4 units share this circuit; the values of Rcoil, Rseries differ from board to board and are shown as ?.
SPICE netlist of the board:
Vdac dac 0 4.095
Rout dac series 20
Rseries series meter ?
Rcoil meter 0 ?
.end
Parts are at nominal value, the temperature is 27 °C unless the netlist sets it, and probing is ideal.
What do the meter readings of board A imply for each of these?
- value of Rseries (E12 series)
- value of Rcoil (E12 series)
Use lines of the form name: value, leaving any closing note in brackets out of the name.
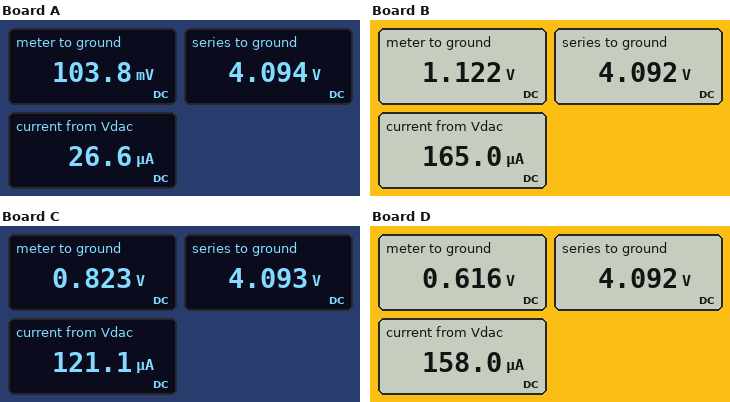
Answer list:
value of Rseries: 150 kΩ
value of Rcoil: 3.9 kΩ
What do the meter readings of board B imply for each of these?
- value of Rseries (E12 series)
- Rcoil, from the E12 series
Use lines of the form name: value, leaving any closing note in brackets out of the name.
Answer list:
value of Rseries: 18 kΩ
Rcoil, from the E12 series: 6.8 kΩ
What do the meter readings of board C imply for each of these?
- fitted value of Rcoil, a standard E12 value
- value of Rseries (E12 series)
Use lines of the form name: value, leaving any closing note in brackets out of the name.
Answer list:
fitted value of Rcoil, a standard E12 value: 6.8 kΩ
value of Rseries: 27 kΩ
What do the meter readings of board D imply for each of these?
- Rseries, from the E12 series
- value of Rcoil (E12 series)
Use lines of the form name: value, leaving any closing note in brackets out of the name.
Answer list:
Rseries, from the E12 series: 22 kΩ
value of Rcoil: 3.9 kΩ
